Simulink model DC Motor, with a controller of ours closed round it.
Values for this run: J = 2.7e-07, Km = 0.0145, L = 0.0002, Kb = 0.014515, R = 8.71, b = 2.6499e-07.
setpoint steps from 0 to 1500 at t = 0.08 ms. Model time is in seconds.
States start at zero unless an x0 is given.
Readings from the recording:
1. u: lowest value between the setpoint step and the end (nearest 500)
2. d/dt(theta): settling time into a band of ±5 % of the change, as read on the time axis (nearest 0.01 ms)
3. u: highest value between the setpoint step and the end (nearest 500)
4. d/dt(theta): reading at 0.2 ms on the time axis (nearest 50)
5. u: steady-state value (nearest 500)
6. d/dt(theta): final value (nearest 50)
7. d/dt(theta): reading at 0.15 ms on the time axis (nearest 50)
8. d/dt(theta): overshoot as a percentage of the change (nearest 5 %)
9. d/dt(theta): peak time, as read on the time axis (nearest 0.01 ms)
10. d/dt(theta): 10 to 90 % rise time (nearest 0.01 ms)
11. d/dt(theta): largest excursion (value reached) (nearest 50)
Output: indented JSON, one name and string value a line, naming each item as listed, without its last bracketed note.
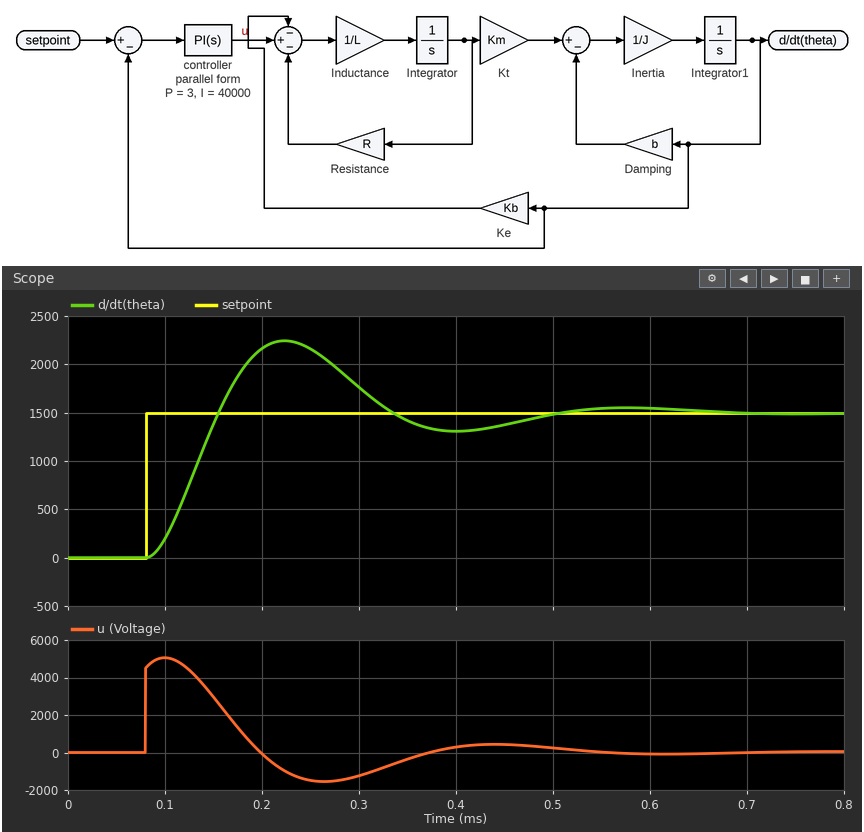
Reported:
{
  "u: lowest value between the setpoint step and the end": "-1500",
  "d/dt(theta): settling time into a band of ±5 % of the change, as read on the time axis": "0.47 ms",
  "u: highest value between the setpoint step and the end": "5000",
  "d/dt(theta): reading at 0.2 ms on the time axis": "2150",
  "u: steady-state value": "0",
  "d/dt(theta): final value": "1500",
  "d/dt(theta): reading at 0.15 ms on the time axis": "1400",
  "d/dt(theta): overshoot as a percentage of the change": "50 %",
  "d/dt(theta): peak time, as read on the time axis": "0.22 ms",
  "d/dt(theta): 10 to 90 % rise time": "0.05 ms",
  "d/dt(theta): largest excursion (value reached)": "2250"
}
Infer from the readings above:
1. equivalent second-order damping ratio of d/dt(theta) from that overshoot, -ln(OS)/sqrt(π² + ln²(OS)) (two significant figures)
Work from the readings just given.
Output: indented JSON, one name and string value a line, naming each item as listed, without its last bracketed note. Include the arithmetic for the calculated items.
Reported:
{
  "equivalent second-order damping ratio of d/dt(theta) from that overshoot, -ln(OS)/sqrt(π² + ln²(OS))": "ln(0.5) = -0.693; 0.693 / sqrt(9.870 + 0.480) = 0.22"
}
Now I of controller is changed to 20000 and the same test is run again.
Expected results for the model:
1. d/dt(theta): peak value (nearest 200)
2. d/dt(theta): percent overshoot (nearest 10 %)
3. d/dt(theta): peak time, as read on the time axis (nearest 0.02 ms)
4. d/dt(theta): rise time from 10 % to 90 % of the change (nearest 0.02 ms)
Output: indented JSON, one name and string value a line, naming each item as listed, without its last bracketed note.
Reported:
{
  "d/dt(theta): peak value": "2000",
  "d/dt(theta): percent overshoot": "30 %",
  "d/dt(theta): peak time, as read on the time axis": "0.24 ms",
  "d/dt(theta): rise time from 10 % to 90 % of the change": "0.06 ms"
}
